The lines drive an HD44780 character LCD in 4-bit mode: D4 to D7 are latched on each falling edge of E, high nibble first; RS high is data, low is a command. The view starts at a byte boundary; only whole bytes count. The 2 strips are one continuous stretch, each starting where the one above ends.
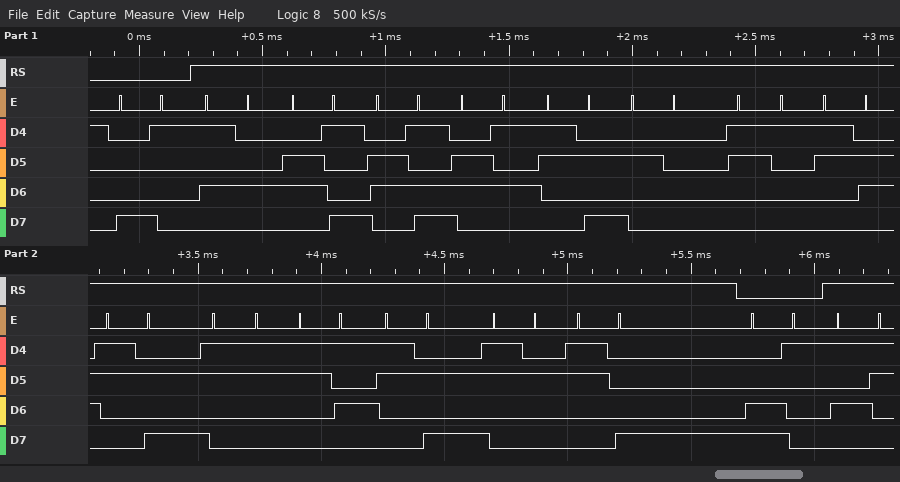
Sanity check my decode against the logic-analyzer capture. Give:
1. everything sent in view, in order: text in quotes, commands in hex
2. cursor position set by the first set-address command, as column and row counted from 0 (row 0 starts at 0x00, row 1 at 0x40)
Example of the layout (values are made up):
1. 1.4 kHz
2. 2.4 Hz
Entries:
1. 0x81 "Time: 16:35:28" 0xC1 "S"
2. column 1, row 0
